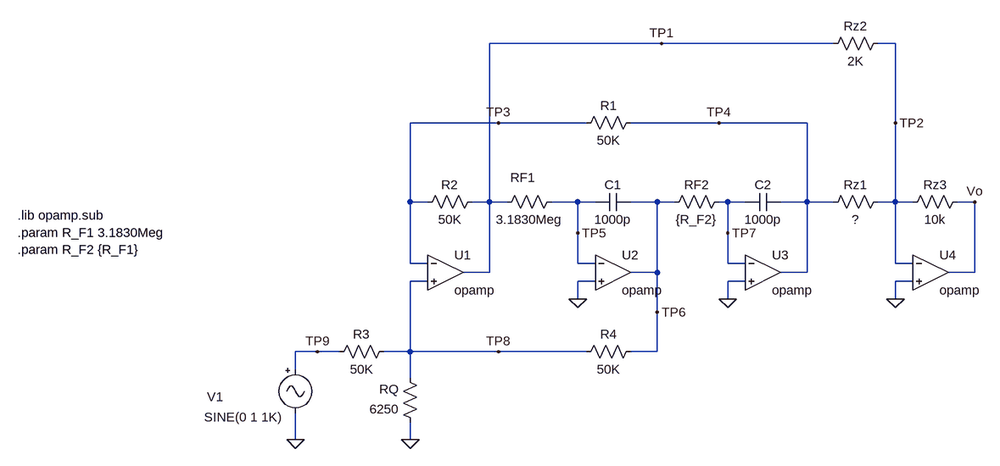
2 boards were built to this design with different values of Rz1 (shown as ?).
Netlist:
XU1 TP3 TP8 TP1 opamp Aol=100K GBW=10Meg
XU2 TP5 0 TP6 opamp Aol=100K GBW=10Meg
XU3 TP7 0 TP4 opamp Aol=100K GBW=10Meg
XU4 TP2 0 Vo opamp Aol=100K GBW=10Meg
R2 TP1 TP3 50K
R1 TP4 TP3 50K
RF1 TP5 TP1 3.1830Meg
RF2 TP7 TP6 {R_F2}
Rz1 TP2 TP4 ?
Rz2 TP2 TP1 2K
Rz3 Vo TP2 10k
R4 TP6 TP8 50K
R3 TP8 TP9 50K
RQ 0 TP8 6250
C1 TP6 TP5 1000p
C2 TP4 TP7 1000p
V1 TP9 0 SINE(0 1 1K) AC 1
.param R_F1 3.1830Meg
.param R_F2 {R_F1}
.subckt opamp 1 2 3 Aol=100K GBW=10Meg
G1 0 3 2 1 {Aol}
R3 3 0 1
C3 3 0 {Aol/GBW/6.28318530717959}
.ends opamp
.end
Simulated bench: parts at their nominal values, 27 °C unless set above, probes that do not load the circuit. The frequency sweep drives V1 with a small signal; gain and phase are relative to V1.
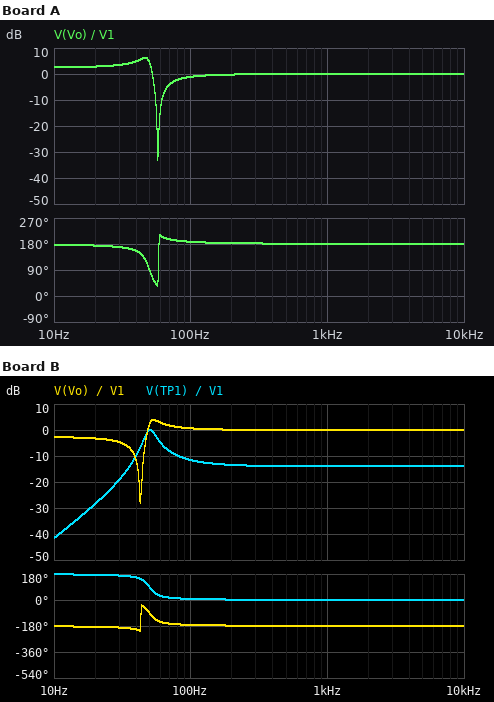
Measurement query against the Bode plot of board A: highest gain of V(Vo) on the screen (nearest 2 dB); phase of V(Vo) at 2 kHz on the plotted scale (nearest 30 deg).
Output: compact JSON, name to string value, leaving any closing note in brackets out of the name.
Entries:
{"highest gain of V(Vo) on the screen": "6 dB", "phase of V(Vo) at 2 kHz on the plotted scale": "180 deg"}
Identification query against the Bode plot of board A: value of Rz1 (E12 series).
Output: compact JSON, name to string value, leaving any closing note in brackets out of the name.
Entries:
{"value of Rz1": "1.5 kΩ"}
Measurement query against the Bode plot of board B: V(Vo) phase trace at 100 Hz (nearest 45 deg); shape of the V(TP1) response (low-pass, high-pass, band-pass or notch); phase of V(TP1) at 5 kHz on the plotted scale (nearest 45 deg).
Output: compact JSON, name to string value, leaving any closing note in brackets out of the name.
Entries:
{"V(Vo) phase trace at 100 Hz": "-180 deg", "shape of the V(TP1) response": "high-pass", "phase of V(TP1) at 5 kHz on the plotted scale": "0 deg"}
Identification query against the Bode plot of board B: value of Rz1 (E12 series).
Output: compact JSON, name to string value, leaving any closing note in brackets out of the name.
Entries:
{"value of Rz1": "2.7 kΩ"}
